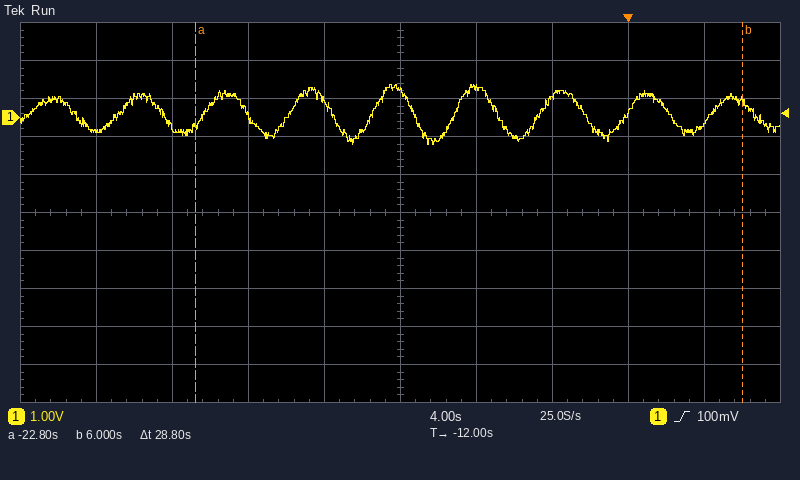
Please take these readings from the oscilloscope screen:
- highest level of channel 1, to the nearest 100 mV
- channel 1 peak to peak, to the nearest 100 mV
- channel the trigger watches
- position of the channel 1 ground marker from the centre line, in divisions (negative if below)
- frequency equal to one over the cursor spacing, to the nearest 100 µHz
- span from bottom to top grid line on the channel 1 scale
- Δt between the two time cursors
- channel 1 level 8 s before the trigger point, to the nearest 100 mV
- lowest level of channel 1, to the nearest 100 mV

900 mV
1.6 V
channel 1
+2.5 div
34.7 mHz
10 V
28.8 s
800 mV
-700 mV
